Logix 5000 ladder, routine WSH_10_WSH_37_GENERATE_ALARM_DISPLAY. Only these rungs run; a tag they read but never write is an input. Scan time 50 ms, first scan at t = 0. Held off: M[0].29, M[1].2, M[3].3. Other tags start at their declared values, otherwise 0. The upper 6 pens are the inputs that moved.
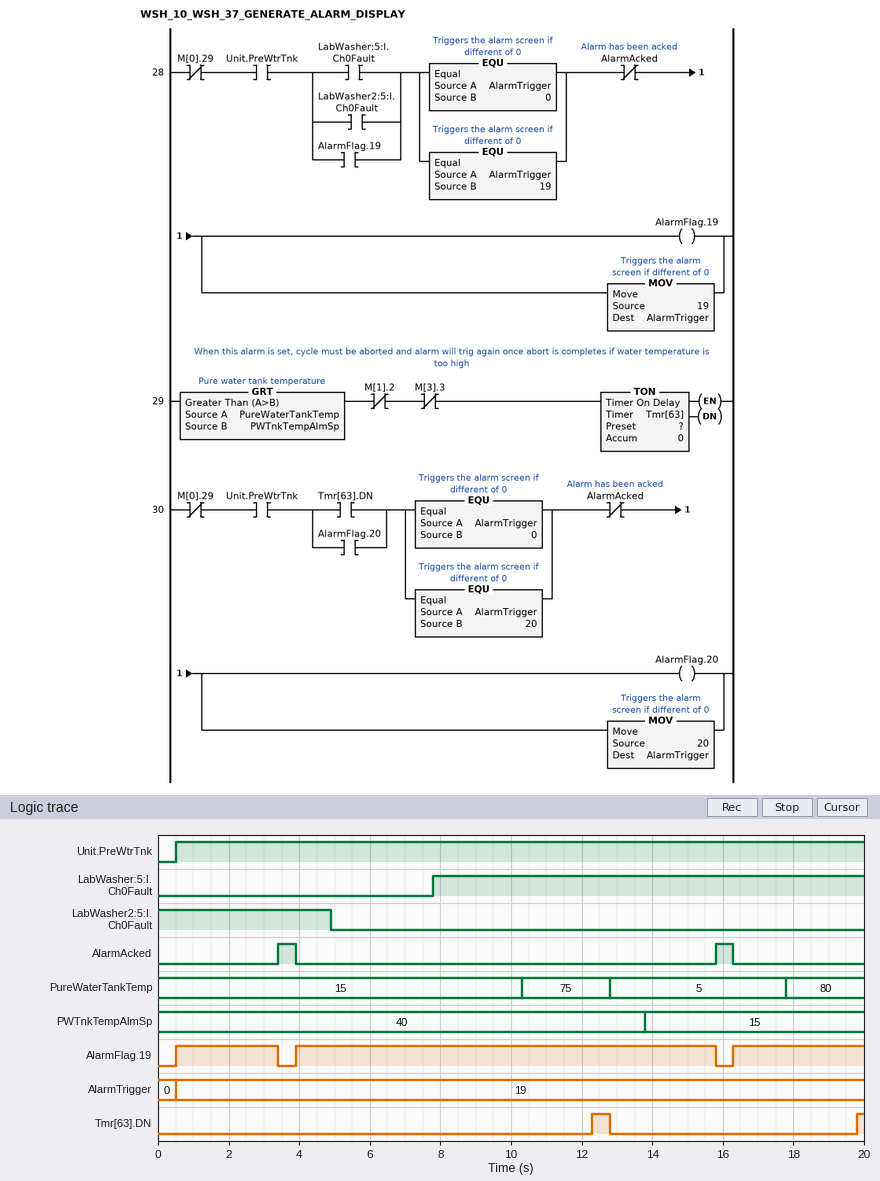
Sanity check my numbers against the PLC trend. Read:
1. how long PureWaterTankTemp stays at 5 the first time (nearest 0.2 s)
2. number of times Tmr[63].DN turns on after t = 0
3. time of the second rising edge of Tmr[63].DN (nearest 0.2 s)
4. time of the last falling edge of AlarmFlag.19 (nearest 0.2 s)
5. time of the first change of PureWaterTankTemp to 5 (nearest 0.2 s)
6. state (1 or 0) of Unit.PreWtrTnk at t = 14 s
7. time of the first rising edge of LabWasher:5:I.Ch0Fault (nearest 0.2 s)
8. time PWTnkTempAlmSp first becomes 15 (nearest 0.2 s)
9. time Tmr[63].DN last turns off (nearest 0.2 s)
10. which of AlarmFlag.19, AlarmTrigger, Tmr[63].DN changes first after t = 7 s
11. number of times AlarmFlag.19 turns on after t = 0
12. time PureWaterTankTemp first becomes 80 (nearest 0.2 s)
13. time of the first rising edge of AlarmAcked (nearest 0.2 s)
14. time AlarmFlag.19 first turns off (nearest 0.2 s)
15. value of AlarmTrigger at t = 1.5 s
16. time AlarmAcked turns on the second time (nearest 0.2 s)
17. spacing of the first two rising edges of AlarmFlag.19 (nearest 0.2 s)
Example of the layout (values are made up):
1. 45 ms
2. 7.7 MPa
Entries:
1. 5.0 s
2. 2
3. 19.8 s
4. 15.8 s
5. 12.8 s
6. 1
7. 7.8 s
8. 13.8 s
9. 12.8 s
10. Tmr[63].DN
11. 3
12. 17.8 s
13. 3.4 s
14. 3.4 s
15. 19
16. 15.8 s
17. 3.4 s
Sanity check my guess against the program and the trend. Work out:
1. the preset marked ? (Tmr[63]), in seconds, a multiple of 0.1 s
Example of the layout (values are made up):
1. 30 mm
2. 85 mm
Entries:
1. 2.0 s
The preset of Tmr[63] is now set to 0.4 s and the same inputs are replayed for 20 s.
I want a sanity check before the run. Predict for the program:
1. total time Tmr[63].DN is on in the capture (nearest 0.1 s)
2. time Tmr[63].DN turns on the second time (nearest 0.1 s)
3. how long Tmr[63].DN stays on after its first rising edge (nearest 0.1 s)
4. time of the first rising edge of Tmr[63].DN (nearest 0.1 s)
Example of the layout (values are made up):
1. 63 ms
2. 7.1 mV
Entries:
1. 3.9 s
2. 18.2 s
3. 2.1 s
4. 10.7 s
